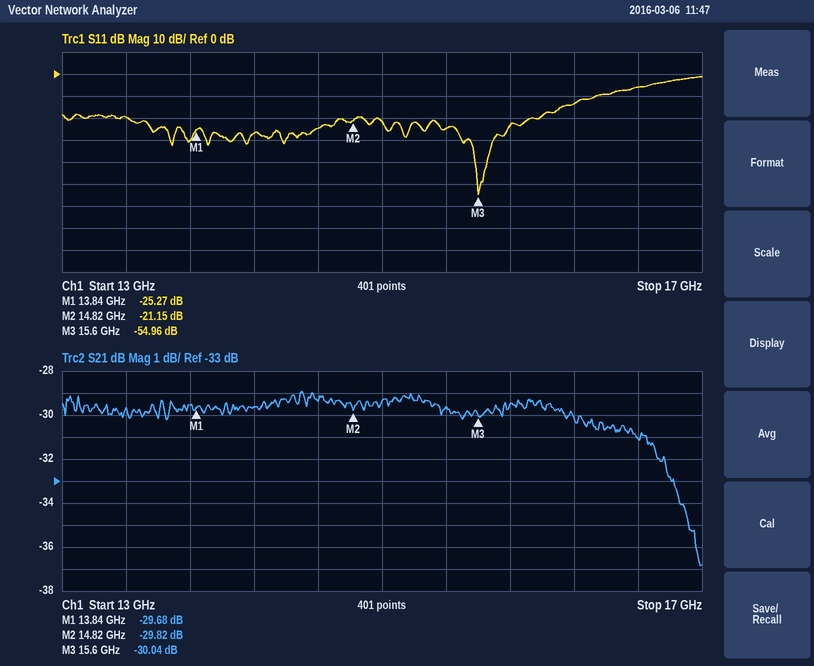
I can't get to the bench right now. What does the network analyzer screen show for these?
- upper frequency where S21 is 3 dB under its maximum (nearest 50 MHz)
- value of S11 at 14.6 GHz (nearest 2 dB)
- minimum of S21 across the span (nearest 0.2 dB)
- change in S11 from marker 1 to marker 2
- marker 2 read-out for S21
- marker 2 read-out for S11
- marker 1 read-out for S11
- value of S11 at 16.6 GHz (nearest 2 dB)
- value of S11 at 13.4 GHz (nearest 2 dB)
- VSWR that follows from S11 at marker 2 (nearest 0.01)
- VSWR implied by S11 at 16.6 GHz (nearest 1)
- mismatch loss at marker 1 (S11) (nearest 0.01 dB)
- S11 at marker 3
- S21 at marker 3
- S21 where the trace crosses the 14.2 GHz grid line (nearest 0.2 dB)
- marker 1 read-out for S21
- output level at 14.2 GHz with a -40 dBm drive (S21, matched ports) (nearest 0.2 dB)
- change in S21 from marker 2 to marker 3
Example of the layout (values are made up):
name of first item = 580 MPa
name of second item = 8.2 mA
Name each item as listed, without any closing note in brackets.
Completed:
upper frequency where S21 is 3 dB under its maximum = 16.70 GHz
value of S11 at 14.6 GHz = -24 dB
minimum of S21 across the span = -36.8 dB
change in S11 from marker 1 to marker 2 = 4.12 dB
marker 2 read-out for S21 = -29.82 dB
marker 2 read-out for S11 = -21.15 dB
marker 1 read-out for S11 = -25.27 dB
value of S11 at 16.6 GHz = -6 dB
value of S11 at 13.4 GHz = -20 dB
VSWR that follows from S11 at marker 2 = 1.19
VSWR implied by S11 at 16.6 GHz = 3
mismatch loss at marker 1 (S11) = 0.01 dB
S11 at marker 3 = -54.96 dB
S21 at marker 3 = -30.04 dB
S21 where the trace crosses the 14.2 GHz grid line = -29.6 dB
marker 1 read-out for S21 = -29.68 dB
output level at 14.2 GHz with a -40 dBm drive (S21, matched ports) = -69.6 dBm
change in S21 from marker 2 to marker 3 = -0.22 dB
